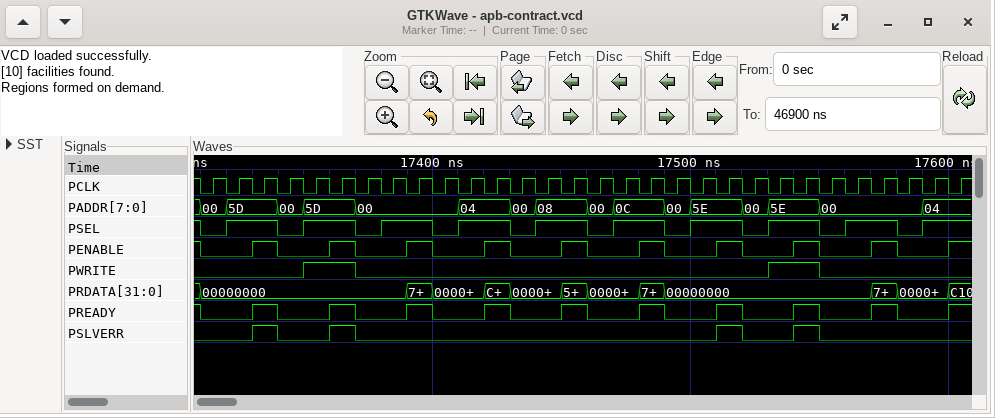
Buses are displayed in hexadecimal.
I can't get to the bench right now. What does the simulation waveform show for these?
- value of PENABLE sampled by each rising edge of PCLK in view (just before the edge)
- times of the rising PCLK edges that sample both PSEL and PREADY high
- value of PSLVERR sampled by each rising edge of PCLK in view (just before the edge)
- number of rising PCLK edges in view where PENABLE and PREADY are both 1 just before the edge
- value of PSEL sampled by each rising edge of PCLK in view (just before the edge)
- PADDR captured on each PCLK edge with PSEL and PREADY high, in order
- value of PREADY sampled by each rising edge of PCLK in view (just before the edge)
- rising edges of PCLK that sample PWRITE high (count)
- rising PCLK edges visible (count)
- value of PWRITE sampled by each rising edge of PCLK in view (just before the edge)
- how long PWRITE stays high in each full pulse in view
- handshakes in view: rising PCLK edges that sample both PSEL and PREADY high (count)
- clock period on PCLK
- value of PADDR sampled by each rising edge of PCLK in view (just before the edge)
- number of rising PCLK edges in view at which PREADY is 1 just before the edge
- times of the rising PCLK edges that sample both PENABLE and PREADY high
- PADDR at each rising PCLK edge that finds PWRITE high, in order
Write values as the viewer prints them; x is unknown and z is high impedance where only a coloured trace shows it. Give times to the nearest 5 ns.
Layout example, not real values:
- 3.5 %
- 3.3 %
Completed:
- 0 0 1 0 0 1 0 0 1 0 0 1 0 0 1 0 0 1 0 0 1 0 0 1 0 0 1 0 0 1
- 17335 ns, 17365 ns, 17395 ns, 17425 ns, 17455 ns, 17485 ns, 17515 ns, 17545 ns, 17575 ns, 17605 ns
- 0 0 1 0 0 1 0 0 0 0 0 0 0 0 0 0 0 0 0 0 1 0 0 1 0 0 0 0 0 0
- 10
- 0 1 1 0 1 1 0 1 1 0 1 1 0 1 1 0 1 1 0 1 1 0 1 1 0 1 1 0 1 1
- 5D, 5D, 00, 04, 08, 0C, 5E, 5E, 00, 04
- 0 0 1 0 0 1 0 0 1 0 0 1 0 0 1 0 0 1 0 0 1 0 0 1 0 0 1 0 0 1
- 4
- 30
- 0 0 0 0 1 1 0 0 0 0 0 0 0 0 0 0 0 0 0 0 0 0 1 1 0 0 0 0 0 0
- 20 ns, 20 ns
- 10
- 10 ns
- 00, 5D, 5D, 00, 5D, 5D, 00, 00, 00, 00, 04, 04, 00, 08, 08, 00, 0C, 0C, 00, 5E, 5E, 00, 5E, 5E, 00, 00, 00, 00, 04, 04
- 10
- 17335 ns, 17365 ns, 17395 ns, 17425 ns, 17455 ns, 17485 ns, 17515 ns, 17545 ns, 17575 ns, 17605 ns
- 5D, 5D, 5E, 5E
